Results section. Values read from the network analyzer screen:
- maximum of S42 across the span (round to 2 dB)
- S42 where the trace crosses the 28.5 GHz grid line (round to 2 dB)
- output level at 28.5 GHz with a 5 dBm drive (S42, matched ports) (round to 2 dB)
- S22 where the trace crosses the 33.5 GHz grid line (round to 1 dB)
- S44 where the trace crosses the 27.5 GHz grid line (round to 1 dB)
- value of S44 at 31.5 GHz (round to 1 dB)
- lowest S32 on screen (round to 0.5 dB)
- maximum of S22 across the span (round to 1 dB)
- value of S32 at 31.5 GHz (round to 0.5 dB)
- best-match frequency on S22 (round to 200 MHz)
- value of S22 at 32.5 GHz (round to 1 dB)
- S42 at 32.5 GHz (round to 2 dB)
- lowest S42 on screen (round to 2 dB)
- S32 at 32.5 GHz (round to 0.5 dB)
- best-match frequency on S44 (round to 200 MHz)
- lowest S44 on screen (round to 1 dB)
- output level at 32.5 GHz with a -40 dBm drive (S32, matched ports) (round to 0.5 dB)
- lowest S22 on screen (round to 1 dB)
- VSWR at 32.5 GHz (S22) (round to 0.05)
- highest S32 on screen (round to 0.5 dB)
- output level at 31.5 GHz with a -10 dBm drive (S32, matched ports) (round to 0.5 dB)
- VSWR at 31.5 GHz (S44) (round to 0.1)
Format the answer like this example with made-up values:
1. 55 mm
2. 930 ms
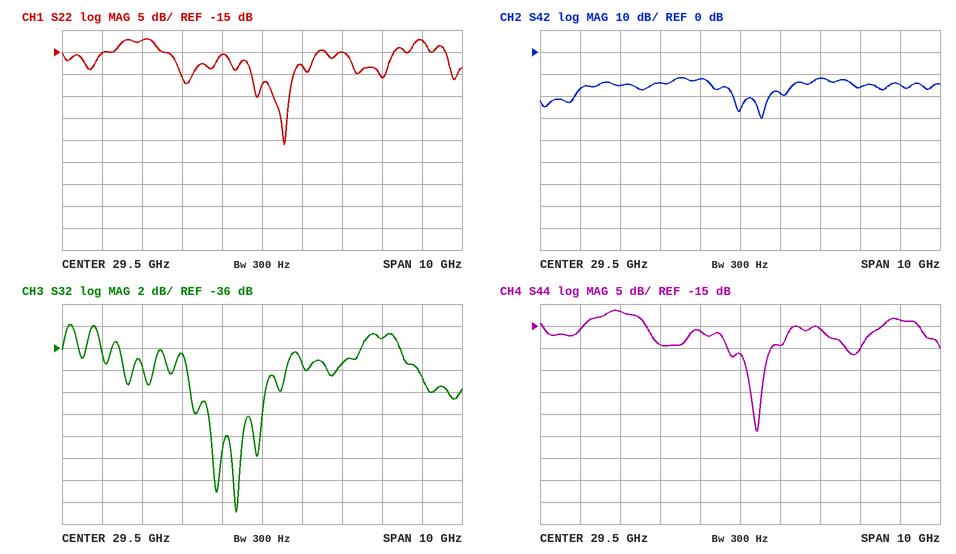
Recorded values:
1. -12 dB
2. -12 dB
3. -8 dBm
4. -12 dB
5. -19 dB
6. -16 dB
7. -51.0 dB
8. -12 dB
9. -37.5 dB
10. 30.0 GHz
11. -21 dB
12. -16 dB
13. -30 dB
14. -35.0 dB
15. 30.0 GHz
16. -39 dB
17. -75.0 dBm
18. -36 dB
19. 1.20
20. -34.0 dB
21. -47.5 dBm
22. 1.4
